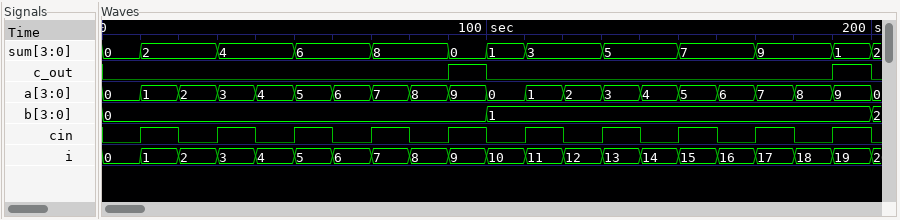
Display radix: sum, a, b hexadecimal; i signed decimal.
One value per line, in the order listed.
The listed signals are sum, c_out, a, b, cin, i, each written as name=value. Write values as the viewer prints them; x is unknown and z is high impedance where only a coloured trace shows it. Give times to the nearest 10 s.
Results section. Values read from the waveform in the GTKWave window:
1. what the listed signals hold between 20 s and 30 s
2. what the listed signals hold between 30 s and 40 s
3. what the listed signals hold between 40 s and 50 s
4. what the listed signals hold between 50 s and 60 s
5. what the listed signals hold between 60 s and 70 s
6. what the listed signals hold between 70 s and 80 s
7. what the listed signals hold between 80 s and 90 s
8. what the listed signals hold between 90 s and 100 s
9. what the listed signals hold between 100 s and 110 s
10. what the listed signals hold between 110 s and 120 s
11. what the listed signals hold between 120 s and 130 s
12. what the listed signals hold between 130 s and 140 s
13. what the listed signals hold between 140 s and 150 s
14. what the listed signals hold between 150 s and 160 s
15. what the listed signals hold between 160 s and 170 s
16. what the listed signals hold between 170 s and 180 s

sum=2, c_out=0, a=2, b=0, cin=0, i=2
sum=4, c_out=0, a=3, b=0, cin=1, i=3
sum=4, c_out=0, a=4, b=0, cin=0, i=4
sum=6, c_out=0, a=5, b=0, cin=1, i=5
sum=6, c_out=0, a=6, b=0, cin=0, i=6
sum=8, c_out=0, a=7, b=0, cin=1, i=7
sum=8, c_out=0, a=8, b=0, cin=0, i=8
sum=0, c_out=1, a=9, b=0, cin=1, i=9
sum=1, c_out=0, a=0, b=1, cin=0, i=10
sum=3, c_out=0, a=1, b=1, cin=1, i=11
sum=3, c_out=0, a=2, b=1, cin=0, i=12
sum=5, c_out=0, a=3, b=1, cin=1, i=13
sum=5, c_out=0, a=4, b=1, cin=0, i=14
sum=7, c_out=0, a=5, b=1, cin=1, i=15
sum=7, c_out=0, a=6, b=1, cin=0, i=16
sum=9, c_out=0, a=7, b=1, cin=1, i=17
